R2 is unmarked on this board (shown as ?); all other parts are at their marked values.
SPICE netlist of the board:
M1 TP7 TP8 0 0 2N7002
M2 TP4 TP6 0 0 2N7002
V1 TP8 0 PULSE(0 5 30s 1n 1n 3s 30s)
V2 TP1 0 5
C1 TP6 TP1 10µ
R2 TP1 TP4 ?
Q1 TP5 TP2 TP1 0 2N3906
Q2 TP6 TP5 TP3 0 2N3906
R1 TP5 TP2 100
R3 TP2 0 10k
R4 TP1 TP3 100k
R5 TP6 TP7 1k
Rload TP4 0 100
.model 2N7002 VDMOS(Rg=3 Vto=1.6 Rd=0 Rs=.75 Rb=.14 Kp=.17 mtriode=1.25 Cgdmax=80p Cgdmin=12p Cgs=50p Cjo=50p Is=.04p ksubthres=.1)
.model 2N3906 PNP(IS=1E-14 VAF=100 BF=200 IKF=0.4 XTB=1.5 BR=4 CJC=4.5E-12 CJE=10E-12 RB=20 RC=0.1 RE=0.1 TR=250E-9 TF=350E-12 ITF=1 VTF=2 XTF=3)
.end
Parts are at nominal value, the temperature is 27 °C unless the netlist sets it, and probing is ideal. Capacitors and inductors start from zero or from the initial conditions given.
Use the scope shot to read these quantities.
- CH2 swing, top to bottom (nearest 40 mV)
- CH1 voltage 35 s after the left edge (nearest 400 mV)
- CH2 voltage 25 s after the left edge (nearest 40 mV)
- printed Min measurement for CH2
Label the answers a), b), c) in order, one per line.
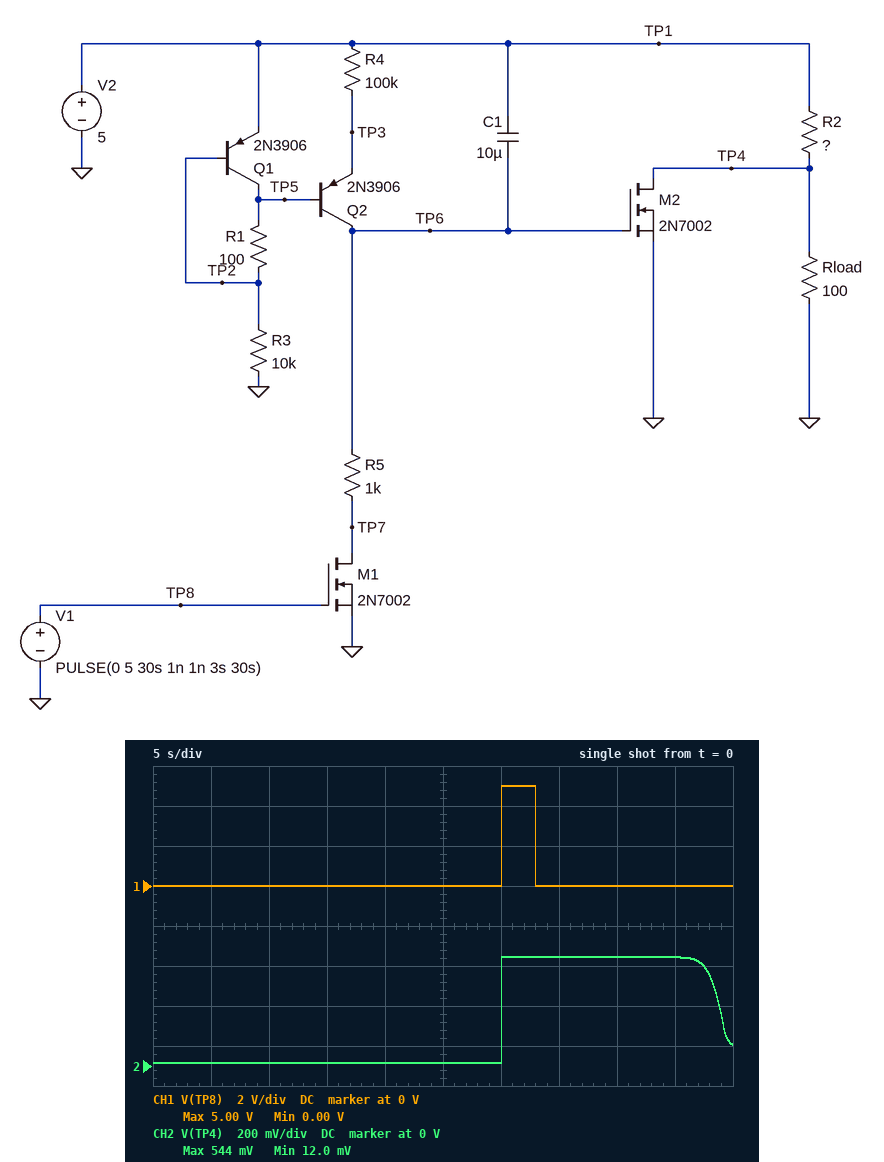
a) 520 mV
b) 0 V
c) 0 V
d) 12.0 mV
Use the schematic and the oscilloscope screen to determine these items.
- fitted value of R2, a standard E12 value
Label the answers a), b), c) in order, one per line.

a) 820 Ω
